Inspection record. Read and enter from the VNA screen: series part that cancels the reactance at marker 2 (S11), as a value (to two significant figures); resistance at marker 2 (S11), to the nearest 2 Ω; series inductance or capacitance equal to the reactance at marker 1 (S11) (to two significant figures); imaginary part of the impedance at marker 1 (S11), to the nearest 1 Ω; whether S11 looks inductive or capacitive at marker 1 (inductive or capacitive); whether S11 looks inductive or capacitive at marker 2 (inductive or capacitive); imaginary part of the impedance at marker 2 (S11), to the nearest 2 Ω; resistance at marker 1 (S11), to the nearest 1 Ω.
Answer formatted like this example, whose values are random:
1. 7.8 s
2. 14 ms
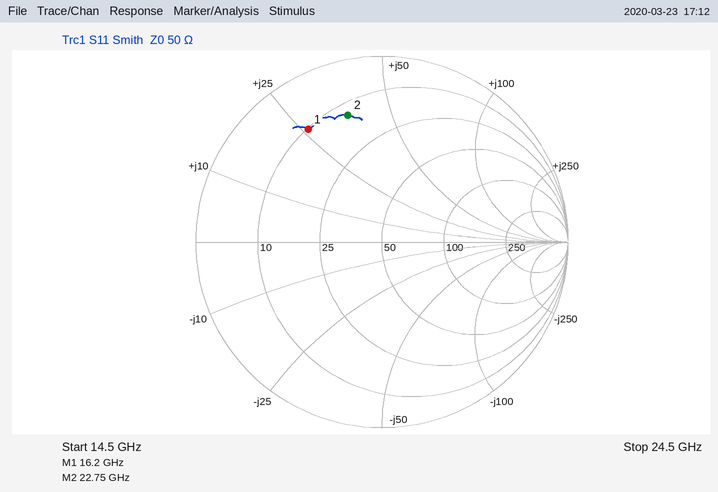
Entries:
1. 190 fF
2. 14 Ω
3. 260 pH
4. +26 Ω
5. inductive
6. inductive
7. +36 Ω
8. 10 Ω
